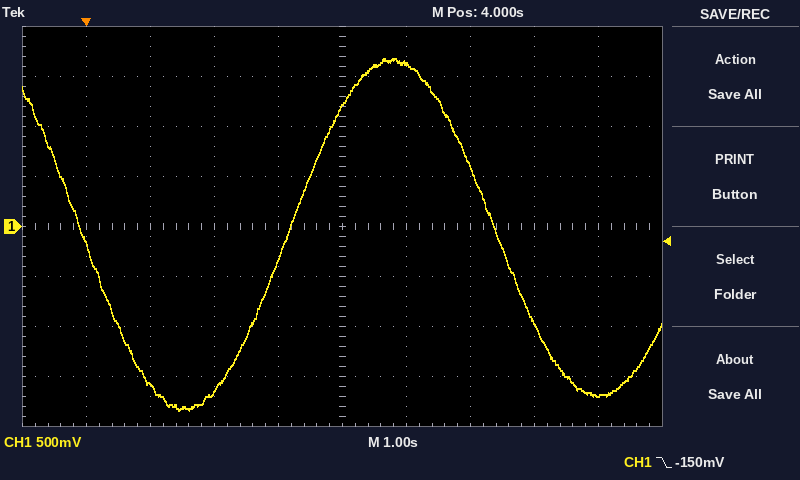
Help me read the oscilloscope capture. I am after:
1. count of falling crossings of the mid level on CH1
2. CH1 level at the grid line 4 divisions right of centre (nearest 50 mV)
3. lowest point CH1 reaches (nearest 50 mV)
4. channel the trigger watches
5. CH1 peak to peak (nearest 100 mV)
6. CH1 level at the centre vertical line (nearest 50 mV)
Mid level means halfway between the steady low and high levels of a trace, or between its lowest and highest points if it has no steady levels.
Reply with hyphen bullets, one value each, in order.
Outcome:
- 2
- -1.70 V
- -1.85 V
- CH1
- 3.50 V
- 1.20 V
